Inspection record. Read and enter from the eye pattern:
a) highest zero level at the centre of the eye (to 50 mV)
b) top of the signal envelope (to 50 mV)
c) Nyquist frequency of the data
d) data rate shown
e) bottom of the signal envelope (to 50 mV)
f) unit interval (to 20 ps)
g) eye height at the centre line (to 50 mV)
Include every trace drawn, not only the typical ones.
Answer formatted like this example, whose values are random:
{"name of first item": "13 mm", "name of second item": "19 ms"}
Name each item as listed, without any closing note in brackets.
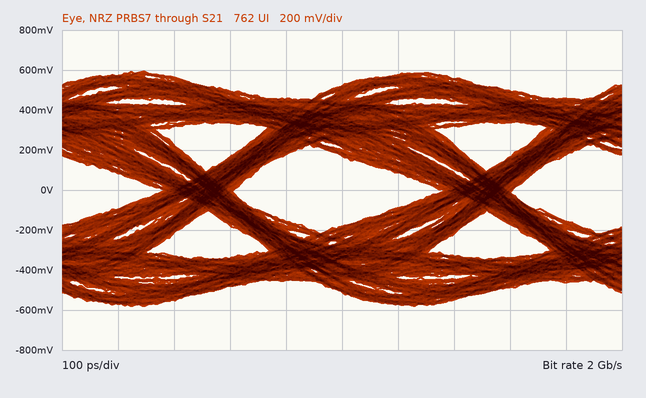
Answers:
{"highest zero level at the centre of the eye": "-200 mV", "top of the signal envelope": "600 mV", "Nyquist frequency of the data": "1 GHz", "data rate shown": "2 Gb/s", "bottom of the signal envelope": "-600 mV", "unit interval": "500 ps", "eye height at the centre line": "350 mV"}
